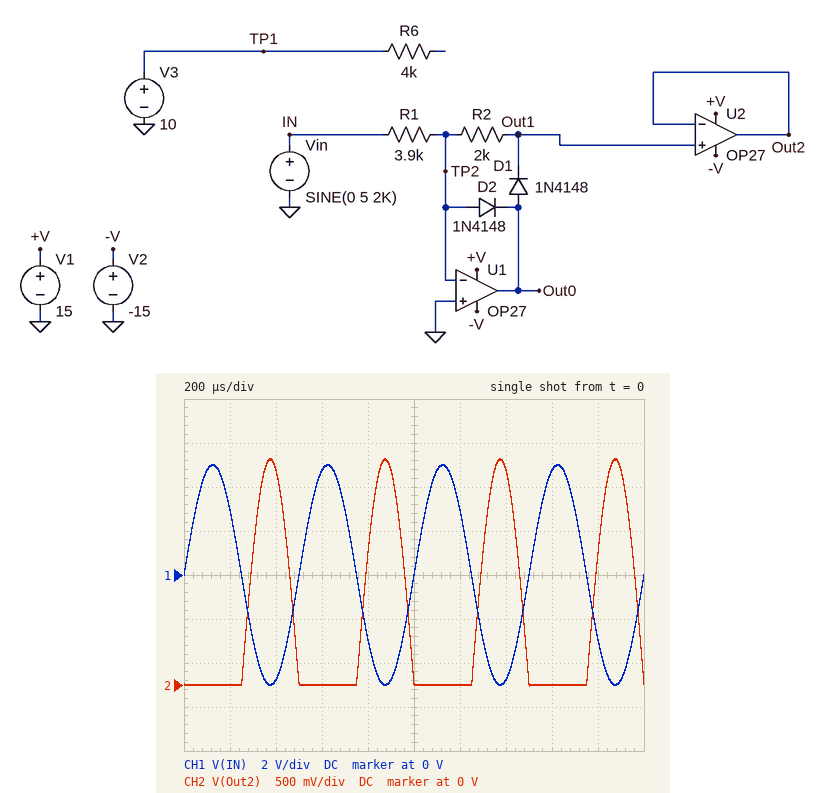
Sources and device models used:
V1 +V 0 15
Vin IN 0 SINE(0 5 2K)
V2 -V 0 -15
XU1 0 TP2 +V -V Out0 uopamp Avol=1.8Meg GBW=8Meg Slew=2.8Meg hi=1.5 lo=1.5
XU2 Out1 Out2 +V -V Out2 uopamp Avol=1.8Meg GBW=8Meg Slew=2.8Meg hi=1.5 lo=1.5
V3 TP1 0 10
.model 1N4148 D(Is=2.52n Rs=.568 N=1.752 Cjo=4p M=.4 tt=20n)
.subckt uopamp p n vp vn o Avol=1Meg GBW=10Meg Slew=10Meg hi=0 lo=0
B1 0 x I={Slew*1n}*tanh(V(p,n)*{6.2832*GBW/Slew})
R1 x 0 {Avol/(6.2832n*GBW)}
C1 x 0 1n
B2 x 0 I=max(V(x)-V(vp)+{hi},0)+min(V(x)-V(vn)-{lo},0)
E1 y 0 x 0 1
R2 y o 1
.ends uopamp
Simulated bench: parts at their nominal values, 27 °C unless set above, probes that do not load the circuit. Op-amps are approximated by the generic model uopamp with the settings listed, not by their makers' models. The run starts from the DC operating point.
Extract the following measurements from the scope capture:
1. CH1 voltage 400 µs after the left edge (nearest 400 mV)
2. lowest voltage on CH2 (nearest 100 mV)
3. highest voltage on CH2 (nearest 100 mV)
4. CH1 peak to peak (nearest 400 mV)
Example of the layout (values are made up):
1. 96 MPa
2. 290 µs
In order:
1. -4.8 V
2. 0 V
3. 2.6 V
4. 10.0 V
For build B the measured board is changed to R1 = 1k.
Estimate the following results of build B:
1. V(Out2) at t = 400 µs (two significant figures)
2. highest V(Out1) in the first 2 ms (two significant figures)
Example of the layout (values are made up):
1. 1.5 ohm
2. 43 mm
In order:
1. 9.5 V
2. 10 V
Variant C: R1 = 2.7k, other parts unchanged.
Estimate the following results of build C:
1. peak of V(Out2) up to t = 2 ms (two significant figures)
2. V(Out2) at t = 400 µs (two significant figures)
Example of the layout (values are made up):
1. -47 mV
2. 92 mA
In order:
1. 3.7 V
2. 3.5 V
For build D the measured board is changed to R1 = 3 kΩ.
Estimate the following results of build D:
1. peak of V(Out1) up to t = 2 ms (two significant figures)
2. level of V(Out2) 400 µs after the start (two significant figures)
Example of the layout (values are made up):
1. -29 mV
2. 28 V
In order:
1. 3.3 V
2. 3.2 V
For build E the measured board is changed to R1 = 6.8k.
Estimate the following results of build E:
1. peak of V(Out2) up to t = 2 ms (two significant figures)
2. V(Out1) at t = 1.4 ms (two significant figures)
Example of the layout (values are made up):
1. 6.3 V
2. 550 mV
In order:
1. 1.5 V
2. 1.4 V
